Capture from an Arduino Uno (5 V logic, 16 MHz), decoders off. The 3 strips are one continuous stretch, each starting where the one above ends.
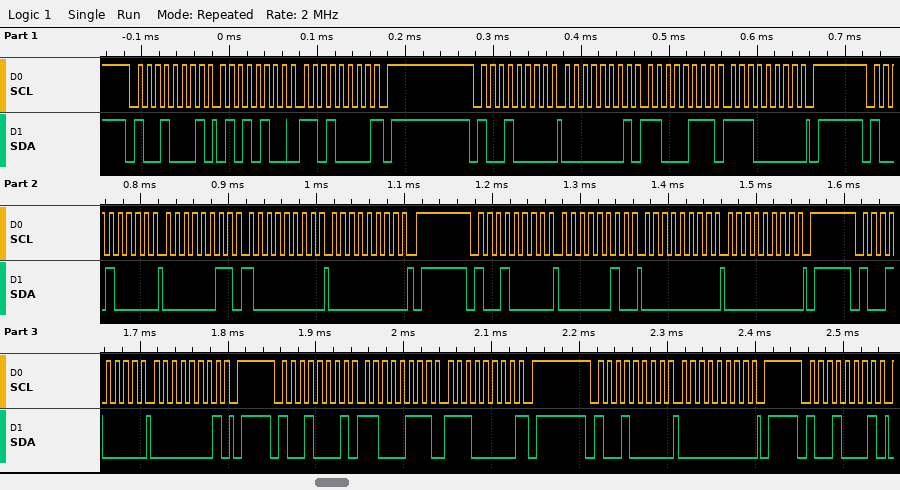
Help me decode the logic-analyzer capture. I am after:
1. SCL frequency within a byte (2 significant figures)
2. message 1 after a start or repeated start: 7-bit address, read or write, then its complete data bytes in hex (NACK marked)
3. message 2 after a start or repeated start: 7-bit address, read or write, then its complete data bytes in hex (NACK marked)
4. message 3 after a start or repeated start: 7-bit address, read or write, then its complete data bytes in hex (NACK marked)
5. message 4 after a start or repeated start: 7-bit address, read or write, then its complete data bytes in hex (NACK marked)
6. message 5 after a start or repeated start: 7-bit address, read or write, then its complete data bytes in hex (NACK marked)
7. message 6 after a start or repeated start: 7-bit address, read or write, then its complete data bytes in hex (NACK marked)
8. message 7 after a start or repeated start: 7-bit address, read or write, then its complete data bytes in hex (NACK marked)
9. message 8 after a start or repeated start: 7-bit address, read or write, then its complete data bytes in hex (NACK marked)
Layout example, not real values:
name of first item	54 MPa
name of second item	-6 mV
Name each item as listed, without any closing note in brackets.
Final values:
SCL frequency within a byte	100 kHz
message 1 after a start or repeated start: 7-bit address, read or write, then its complete data bytes in hex	0x48 read: 54 D0 NACK
message 2 after a start or repeated start: 7-bit address, read or write, then its complete data bytes in hex	0x48 write: 01 C7 E0
message 3 after a start or repeated start: 7-bit address, read or write, then its complete data bytes in hex	0x48 write: 03 80 00
message 4 after a start or repeated start: 7-bit address, read or write, then its complete data bytes in hex	0x48 write: 02 00 00
message 5 after a start or repeated start: 7-bit address, read or write, then its complete data bytes in hex	0x48 write: 01
message 6 after a start or repeated start: 7-bit address, read or write, then its complete data bytes in hex	0x48 read: C7 E0 NACK
message 7 after a start or repeated start: 7-bit address, read or write, then its complete data bytes in hex	0x48 write: 00
message 8 after a start or repeated start: 7-bit address, read or write, then its complete data bytes in hex	0x48 read
